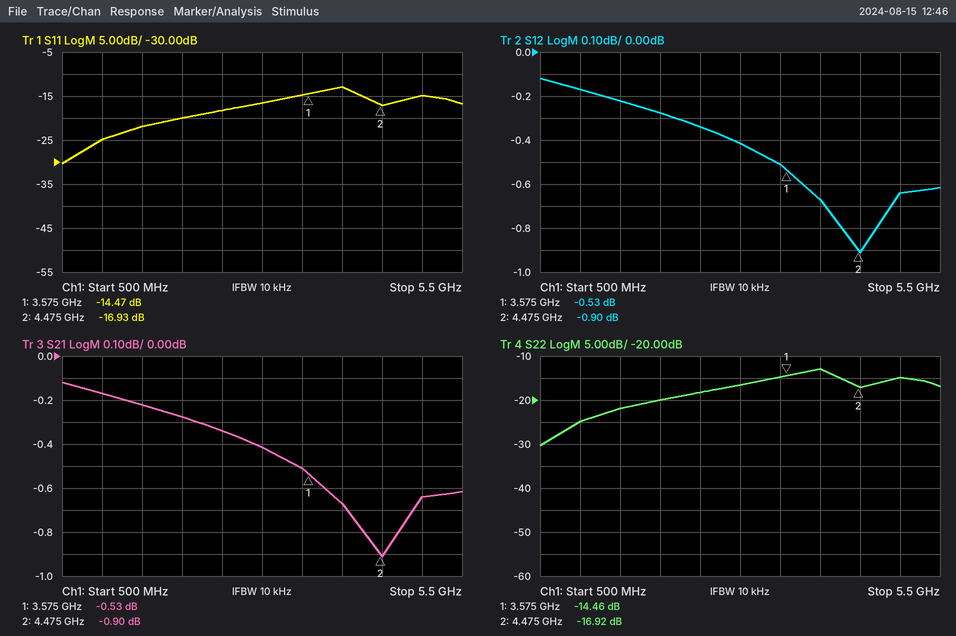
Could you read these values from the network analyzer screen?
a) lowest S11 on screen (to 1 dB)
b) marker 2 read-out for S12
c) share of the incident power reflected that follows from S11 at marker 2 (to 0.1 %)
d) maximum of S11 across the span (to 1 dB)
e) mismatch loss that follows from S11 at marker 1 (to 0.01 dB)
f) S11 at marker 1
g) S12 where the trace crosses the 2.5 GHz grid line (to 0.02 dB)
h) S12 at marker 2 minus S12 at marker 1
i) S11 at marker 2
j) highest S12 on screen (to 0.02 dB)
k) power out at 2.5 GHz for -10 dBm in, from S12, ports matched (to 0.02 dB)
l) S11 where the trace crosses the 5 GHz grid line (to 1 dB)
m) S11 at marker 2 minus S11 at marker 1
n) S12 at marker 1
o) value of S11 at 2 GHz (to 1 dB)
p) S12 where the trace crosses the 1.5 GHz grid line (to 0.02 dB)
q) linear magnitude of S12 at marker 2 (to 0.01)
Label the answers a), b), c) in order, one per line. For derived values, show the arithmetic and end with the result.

a) -30 dB
b) -0.90 dB
c) 10^(-16.93/10) ≈ 2.0 %
d) -13 dB
e) −10 log10(1 − 10^(-14.47/10)) ≈ 0.16 dB
f) -14.47 dB
g) -0.34 dB
h) -0.9 − (-0.53) = -0.37 dB
i) -16.93 dB
j) -0.12 dB
k) -10 dBm + (-0.34 dB) = -10.34 dBm
l) -15 dB
m) -16.93 − (-14.47) = -2.46 dB
n) -0.53 dB
o) -20 dB
p) -0.22 dB
q) 10^(-0.9/20) ≈ 0.90
